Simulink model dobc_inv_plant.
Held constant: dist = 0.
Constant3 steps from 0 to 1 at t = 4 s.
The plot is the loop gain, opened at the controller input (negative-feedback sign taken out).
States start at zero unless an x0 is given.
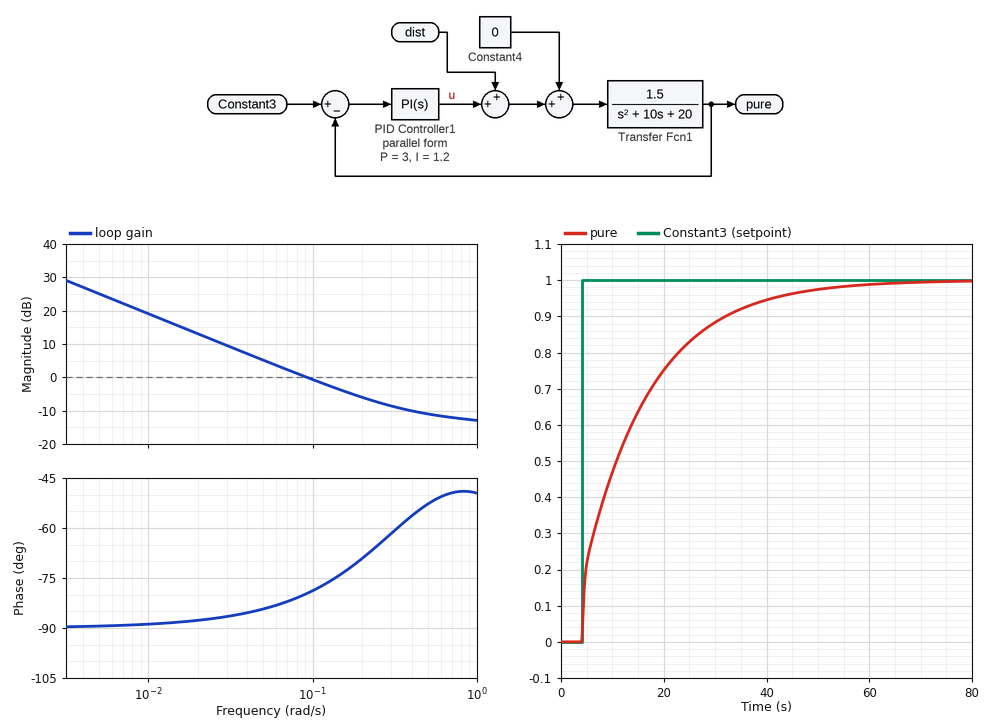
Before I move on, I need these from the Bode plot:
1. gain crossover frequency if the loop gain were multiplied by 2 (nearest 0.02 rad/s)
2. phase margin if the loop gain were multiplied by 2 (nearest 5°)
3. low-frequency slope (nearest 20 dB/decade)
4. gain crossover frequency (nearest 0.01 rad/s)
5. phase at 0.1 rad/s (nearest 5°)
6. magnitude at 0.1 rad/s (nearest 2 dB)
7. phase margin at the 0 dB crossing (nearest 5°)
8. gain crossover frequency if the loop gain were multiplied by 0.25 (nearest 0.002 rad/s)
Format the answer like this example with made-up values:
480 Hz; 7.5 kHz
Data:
0.20 rad/s; 110°; -20 dB/decade; 0.09 rad/s; -80°; 0 dB; 100°; 0.022 rad/s
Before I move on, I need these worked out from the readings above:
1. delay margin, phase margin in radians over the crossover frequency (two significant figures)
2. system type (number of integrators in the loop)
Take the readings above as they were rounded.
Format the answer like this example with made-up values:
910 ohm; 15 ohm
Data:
19 s; 1
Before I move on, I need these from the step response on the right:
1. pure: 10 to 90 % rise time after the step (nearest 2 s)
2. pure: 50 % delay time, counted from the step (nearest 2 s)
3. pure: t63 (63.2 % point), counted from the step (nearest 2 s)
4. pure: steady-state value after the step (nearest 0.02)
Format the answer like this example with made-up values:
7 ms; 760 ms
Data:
28 s; 6 s; 10 s; 1.00
